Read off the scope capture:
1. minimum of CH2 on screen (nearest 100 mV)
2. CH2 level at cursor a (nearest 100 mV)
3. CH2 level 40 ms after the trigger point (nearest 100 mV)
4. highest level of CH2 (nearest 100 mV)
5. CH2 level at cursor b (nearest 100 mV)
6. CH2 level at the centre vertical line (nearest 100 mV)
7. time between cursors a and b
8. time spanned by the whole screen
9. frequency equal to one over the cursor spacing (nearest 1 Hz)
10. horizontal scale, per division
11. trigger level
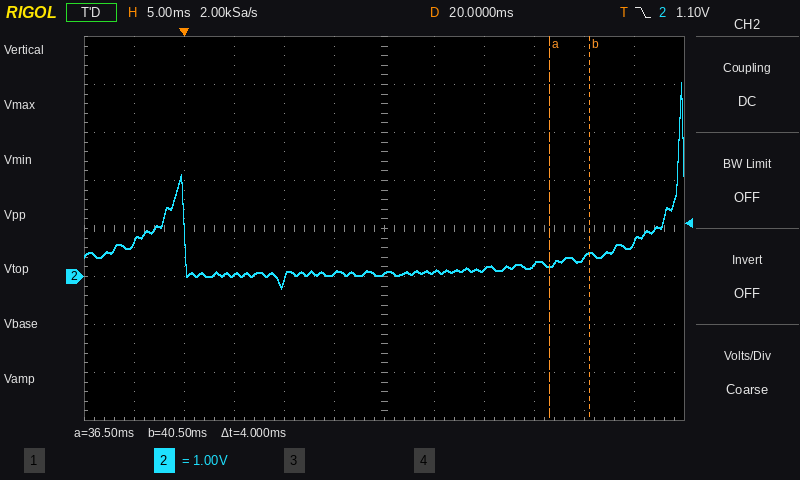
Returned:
-200 mV
200 mV
400 mV
4.0 V
500 mV
100 mV
4 ms
60 ms
250 Hz
5 ms
1.10 V
